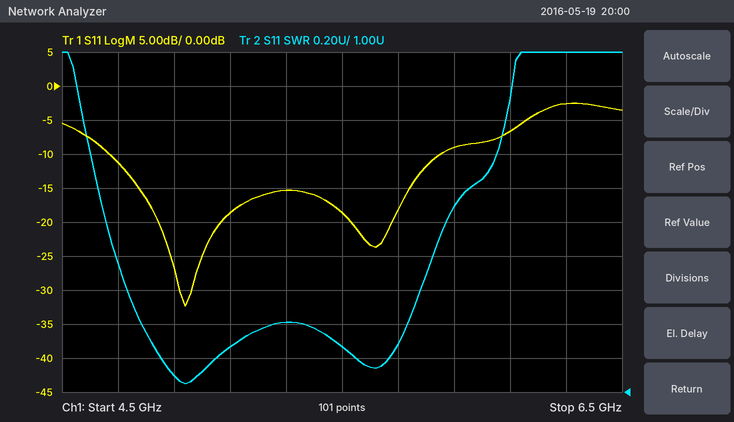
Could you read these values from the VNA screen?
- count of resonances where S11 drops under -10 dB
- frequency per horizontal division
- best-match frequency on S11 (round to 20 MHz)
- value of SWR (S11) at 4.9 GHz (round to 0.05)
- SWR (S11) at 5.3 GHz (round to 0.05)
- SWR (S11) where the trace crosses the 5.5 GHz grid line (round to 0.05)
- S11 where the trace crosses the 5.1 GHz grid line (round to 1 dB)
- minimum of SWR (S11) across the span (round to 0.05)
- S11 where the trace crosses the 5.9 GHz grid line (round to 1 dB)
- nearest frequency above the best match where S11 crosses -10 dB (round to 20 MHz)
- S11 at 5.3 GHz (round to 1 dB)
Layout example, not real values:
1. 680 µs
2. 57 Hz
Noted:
1. 2
2. 200 MHz
3. 4.94 GHz
4. 1.10
5. 1.40
6. 1.25
7. -19 dB
8. 1.05
9. -9 dB
10. 5.86 GHz
11. -15 dB
